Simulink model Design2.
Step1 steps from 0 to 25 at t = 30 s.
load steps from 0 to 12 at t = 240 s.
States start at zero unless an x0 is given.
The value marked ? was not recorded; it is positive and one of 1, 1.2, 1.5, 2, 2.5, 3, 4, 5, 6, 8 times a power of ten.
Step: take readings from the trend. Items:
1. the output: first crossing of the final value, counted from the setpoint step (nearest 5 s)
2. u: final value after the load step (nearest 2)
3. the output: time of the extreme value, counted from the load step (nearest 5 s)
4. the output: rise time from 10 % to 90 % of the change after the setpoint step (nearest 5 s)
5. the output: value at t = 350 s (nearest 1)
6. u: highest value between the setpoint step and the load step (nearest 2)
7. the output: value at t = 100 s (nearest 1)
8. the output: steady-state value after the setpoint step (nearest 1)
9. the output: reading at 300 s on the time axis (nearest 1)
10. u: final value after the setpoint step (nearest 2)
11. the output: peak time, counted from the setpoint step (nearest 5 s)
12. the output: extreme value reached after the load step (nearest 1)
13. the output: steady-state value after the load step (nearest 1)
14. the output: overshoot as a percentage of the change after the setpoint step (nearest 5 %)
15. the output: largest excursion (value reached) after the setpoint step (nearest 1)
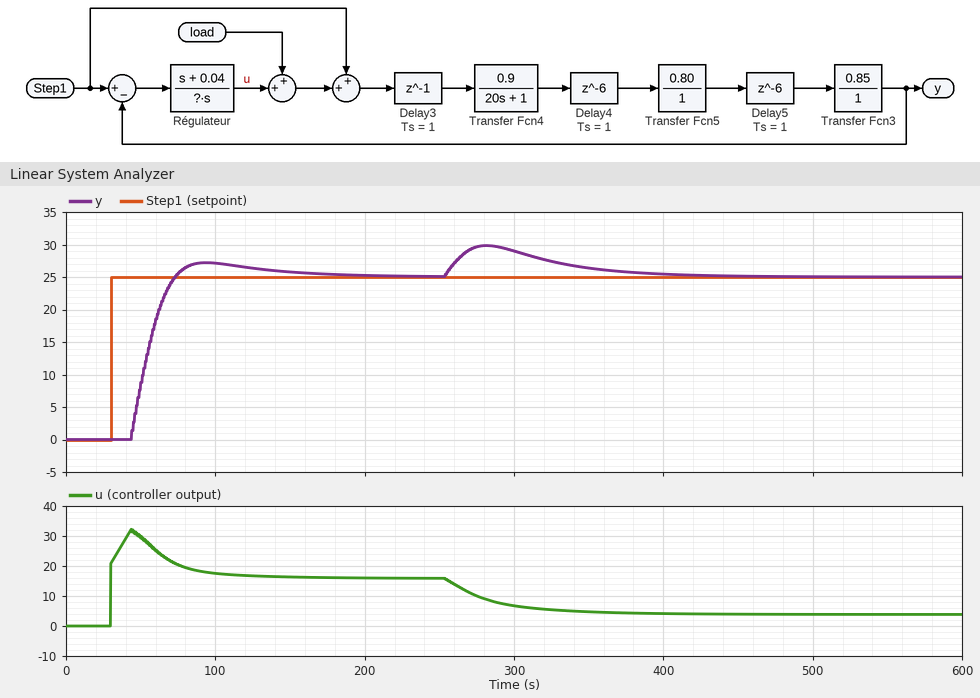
45 s
4
40 s
20 s
26
32
27
25
29
16
65 s
30
25
10 %
27
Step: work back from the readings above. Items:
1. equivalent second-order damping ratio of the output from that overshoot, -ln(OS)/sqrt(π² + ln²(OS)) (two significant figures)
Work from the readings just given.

0.59
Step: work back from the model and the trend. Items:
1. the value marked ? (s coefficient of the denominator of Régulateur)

1.2
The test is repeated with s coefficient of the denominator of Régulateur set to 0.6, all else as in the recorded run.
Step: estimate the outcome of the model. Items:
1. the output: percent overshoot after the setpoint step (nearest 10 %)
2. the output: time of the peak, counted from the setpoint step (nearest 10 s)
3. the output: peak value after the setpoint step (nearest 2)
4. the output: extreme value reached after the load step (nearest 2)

40 %
40 s
34
30
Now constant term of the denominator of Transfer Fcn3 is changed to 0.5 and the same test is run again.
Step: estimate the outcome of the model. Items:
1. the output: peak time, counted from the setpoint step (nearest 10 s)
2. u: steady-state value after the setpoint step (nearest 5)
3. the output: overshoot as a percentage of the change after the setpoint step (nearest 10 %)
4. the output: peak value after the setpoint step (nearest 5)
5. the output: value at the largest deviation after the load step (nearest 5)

40 s
-5
70 %
45
35
